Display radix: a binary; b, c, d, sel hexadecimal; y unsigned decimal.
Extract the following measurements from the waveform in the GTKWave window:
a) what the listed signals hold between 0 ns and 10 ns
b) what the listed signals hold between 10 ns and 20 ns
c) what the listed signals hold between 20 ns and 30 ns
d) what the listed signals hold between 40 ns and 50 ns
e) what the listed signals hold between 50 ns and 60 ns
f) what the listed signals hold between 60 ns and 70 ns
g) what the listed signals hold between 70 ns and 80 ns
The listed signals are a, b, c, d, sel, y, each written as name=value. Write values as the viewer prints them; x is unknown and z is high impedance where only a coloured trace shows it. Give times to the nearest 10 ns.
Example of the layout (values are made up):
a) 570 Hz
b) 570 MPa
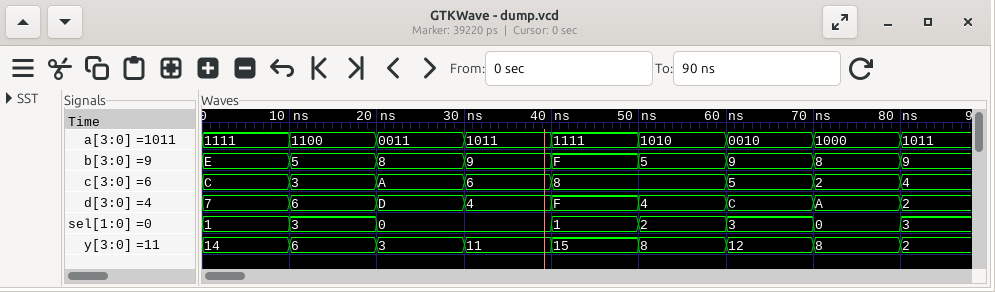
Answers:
a) a=1111, b=E, c=C, d=7, sel=1, y=14
b) a=1100, b=5, c=3, d=6, sel=3, y=6
c) a=0011, b=8, c=A, d=D, sel=0, y=3
d) a=1111, b=F, c=8, d=F, sel=1, y=15
e) a=1010, b=5, c=8, d=4, sel=2, y=8
f) a=0010, b=9, c=5, d=C, sel=3, y=12
g) a=1000, b=8, c=2, d=A, sel=0, y=8
